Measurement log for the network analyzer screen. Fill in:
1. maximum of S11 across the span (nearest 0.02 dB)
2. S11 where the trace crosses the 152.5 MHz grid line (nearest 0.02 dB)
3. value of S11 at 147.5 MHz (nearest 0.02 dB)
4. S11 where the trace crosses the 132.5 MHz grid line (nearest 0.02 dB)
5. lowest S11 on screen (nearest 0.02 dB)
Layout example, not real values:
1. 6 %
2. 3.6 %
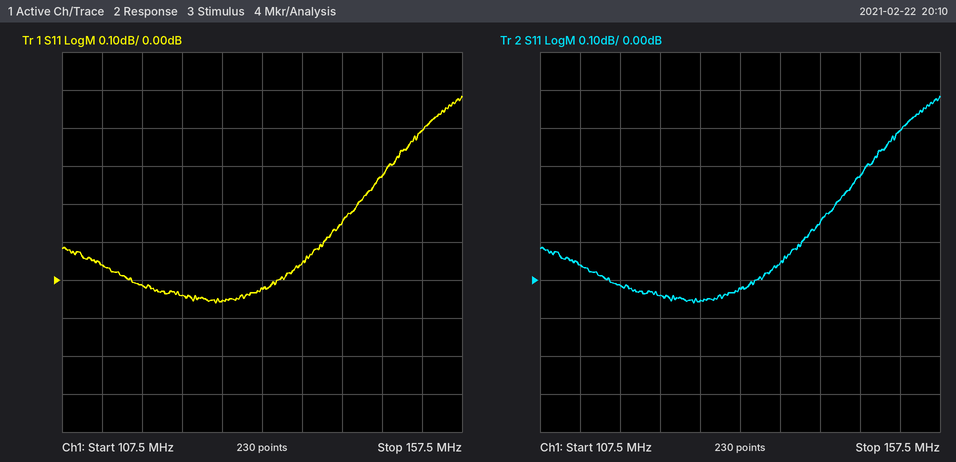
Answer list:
1. 0.48 dB
2. 0.40 dB
3. 0.28 dB
4. -0.02 dB
5. -0.06 dB
